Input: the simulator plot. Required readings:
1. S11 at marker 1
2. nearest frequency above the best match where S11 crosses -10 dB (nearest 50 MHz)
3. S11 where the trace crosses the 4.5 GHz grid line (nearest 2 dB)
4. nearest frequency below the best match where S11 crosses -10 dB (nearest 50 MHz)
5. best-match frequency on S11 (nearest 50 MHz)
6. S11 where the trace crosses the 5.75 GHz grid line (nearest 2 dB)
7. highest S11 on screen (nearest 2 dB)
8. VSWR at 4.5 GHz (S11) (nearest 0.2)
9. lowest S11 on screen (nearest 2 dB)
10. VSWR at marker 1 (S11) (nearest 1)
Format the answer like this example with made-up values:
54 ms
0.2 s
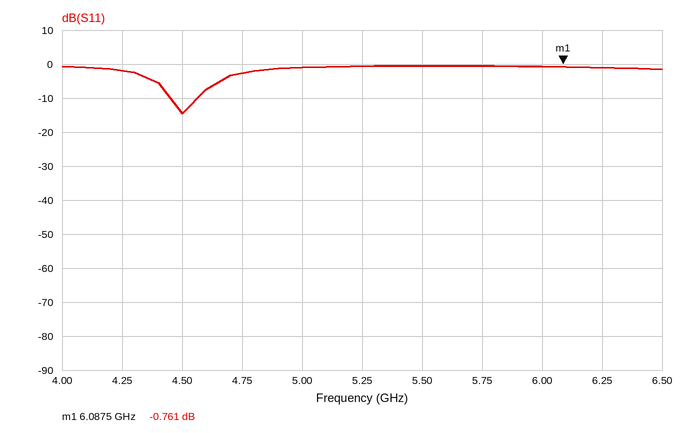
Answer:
-0.761 dB
4.55 GHz
-14 dB
4.45 GHz
4.50 GHz
0 dB
0 dB
1.4
-14 dB
23
